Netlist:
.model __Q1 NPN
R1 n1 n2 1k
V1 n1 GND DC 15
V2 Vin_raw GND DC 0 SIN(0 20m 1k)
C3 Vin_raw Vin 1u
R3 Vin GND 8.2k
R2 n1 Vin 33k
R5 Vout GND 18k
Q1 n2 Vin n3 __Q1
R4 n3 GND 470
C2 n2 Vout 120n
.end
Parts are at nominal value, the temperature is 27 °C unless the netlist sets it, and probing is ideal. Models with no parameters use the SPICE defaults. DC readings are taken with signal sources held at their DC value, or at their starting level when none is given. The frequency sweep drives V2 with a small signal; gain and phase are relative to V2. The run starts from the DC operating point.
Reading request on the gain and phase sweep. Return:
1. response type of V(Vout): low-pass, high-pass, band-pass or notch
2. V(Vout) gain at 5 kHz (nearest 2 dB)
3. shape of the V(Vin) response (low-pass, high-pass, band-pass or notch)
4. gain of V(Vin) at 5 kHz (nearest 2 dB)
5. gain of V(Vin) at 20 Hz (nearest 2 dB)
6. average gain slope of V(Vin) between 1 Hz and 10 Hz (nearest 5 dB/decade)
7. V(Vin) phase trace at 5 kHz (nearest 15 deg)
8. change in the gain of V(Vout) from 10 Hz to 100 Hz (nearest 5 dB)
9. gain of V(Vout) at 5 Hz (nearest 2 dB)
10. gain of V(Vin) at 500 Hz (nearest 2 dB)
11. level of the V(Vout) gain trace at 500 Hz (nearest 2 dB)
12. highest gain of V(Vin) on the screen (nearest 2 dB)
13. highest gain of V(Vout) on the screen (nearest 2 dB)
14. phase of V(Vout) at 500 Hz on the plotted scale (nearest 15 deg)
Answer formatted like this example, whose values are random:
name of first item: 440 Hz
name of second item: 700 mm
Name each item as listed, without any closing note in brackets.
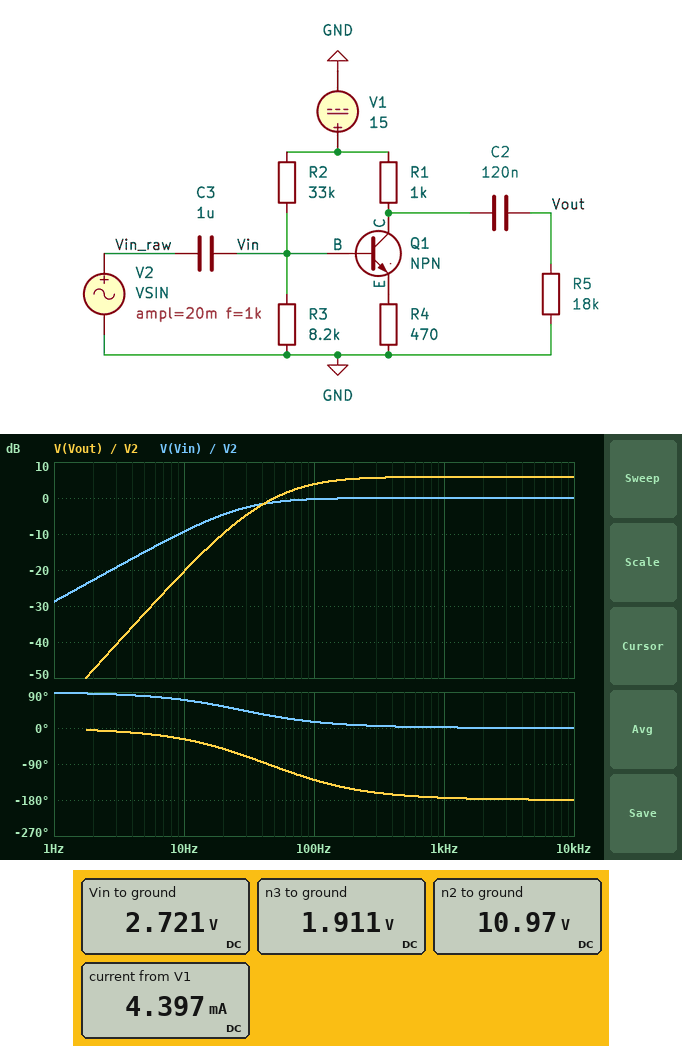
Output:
response type of V(Vout): low-pass, high-pass, band-pass or notch: high-pass
V(Vout) gain at 5 kHz: 6 dB
shape of the V(Vin) response: high-pass
gain of V(Vin) at 5 kHz: 0 dB
gain of V(Vin) at 20 Hz: -4 dB
average gain slope of V(Vin) between 1 Hz and 10 Hz: 20 dB/decade
V(Vin) phase trace at 5 kHz: 0 deg
change in the gain of V(Vout) from 10 Hz to 100 Hz: 25 dB
gain of V(Vout) at 5 Hz: -32 dB
gain of V(Vin) at 500 Hz: 0 dB
level of the V(Vout) gain trace at 500 Hz: 6 dB
highest gain of V(Vin) on the screen: 0 dB
highest gain of V(Vout) on the screen: 6 dB
phase of V(Vout) at 500 Hz on the plotted scale: -165 deg
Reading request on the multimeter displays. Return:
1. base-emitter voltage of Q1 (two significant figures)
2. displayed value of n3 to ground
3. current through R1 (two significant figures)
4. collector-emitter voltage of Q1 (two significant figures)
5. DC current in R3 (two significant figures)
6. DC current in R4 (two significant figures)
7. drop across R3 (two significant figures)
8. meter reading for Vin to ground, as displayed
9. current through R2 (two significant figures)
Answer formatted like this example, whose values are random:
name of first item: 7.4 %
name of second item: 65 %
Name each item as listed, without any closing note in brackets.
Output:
base-emitter voltage of Q1: 810 mV
displayed value of n3 to ground: 1.911 V
current through R1: 4.0 mA
collector-emitter voltage of Q1: 9.1 V
DC current in R3: 330 µA
DC current in R4: 4.1 mA
drop across R3: 2.7 V
meter reading for Vin to ground, as displayed: 2.721 V
current through R2: 370 µA
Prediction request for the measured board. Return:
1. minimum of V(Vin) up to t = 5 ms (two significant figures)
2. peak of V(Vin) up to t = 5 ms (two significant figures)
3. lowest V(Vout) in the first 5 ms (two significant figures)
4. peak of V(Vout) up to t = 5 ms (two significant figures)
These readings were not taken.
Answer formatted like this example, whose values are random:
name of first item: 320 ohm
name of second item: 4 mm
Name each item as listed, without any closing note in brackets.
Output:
minimum of V(Vin) up to t = 5 ms: 2.7 V
peak of V(Vin) up to t = 5 ms: 2.7 V
lowest V(Vout) in the first 5 ms: -39 mV
peak of V(Vout) up to t = 5 ms: 42 mV
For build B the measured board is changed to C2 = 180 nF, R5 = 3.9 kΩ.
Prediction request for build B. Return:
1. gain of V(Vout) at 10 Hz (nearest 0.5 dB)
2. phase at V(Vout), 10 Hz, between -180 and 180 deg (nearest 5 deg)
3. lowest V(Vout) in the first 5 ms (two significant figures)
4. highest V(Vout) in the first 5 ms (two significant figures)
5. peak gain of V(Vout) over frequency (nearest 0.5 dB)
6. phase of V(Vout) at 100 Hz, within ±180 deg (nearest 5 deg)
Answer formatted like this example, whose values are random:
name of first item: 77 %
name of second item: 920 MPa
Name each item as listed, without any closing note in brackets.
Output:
gain of V(Vout) at 10 Hz: -30.0 dB
phase at V(Vout), 10 Hz, between -180 and 180 deg: -25 deg
lowest V(Vout) in the first 5 ms: -33 mV
highest V(Vout) in the first 5 ms: 35 mV
peak gain of V(Vout) over frequency: 4.5 dB
phase of V(Vout) at 100 Hz, within ±180 deg: -105 deg
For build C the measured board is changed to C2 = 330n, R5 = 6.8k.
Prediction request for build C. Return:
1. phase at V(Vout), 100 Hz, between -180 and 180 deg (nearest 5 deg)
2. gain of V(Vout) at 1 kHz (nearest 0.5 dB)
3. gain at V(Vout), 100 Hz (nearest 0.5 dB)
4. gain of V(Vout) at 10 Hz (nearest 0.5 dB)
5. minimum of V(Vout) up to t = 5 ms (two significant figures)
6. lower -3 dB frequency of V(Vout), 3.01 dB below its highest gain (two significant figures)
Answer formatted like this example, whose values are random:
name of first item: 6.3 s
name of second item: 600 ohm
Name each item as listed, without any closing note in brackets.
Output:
phase at V(Vout), 100 Hz, between -180 and 180 deg: -135 deg
gain of V(Vout) at 1 kHz: 5.0 dB
gain at V(Vout), 100 Hz: 3.5 dB
gain of V(Vout) at 10 Hz: -20.0 dB
minimum of V(Vout) up to t = 5 ms: -36 mV
lower -3 dB frequency of V(Vout), 3.01 dB below its highest gain: 72 Hz
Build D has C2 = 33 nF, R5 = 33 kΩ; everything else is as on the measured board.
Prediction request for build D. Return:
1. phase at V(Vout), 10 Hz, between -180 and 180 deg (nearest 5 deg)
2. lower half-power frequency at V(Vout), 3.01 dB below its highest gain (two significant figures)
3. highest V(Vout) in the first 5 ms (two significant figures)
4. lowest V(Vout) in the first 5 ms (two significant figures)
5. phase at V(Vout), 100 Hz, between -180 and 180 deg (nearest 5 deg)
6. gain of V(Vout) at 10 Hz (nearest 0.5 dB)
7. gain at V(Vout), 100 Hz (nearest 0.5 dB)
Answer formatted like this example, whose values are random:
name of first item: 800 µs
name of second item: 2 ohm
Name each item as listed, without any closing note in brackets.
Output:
phase at V(Vout), 10 Hz, between -180 and 180 deg: -25 deg
lower half-power frequency at V(Vout), 3.01 dB below its highest gain: 150 Hz
highest V(Vout) in the first 5 ms: 43 mV
lowest V(Vout) in the first 5 ms: -40 mV
phase at V(Vout), 100 Hz, between -180 and 180 deg: -110 deg
gain of V(Vout) at 10 Hz: -26.5 dB
gain at V(Vout), 100 Hz: 1.0 dB
